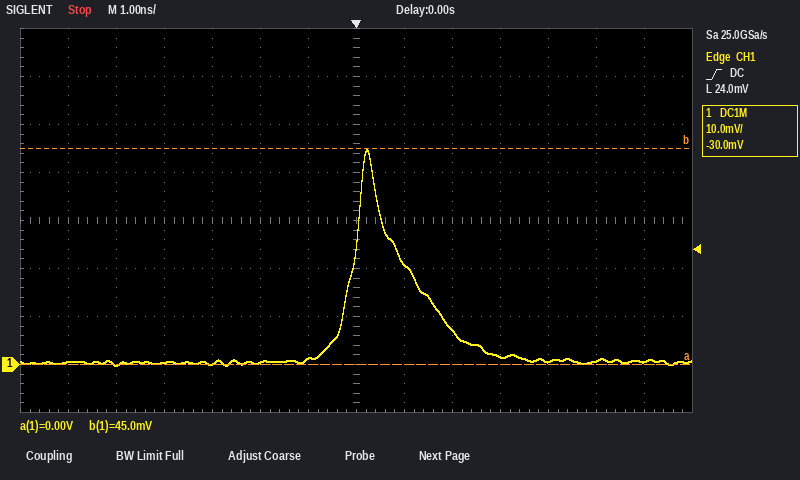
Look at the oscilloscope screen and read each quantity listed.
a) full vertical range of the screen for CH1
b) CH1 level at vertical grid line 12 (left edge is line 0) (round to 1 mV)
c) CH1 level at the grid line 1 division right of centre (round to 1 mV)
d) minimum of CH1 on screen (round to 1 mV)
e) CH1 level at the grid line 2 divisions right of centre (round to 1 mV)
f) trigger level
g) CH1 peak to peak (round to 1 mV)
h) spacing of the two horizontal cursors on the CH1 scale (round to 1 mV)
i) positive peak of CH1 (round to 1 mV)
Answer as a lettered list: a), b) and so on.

a) 80 mV
b) 1 mV
c) 21 mV
d) 0 mV
e) 7 mV
f) 24.0 mV
g) 45 mV
h) 45 mV
i) 45 mV
